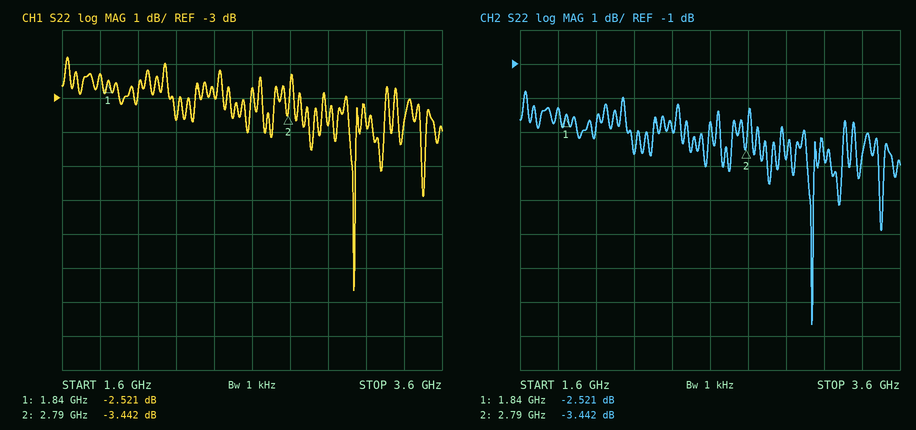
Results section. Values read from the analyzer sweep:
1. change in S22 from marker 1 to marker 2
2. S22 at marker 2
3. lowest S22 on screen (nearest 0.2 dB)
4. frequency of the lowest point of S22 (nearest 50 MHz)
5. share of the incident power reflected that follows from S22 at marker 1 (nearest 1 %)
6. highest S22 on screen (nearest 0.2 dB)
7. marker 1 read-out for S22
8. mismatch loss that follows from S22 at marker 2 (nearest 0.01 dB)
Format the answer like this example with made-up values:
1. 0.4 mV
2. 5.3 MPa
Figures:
1. -0.921 dB
2. -3.442 dB
3. -8.6 dB
4. 3.15 GHz
5. 56 %
6. -1.8 dB
7. -2.521 dB
8. 2.62 dB
